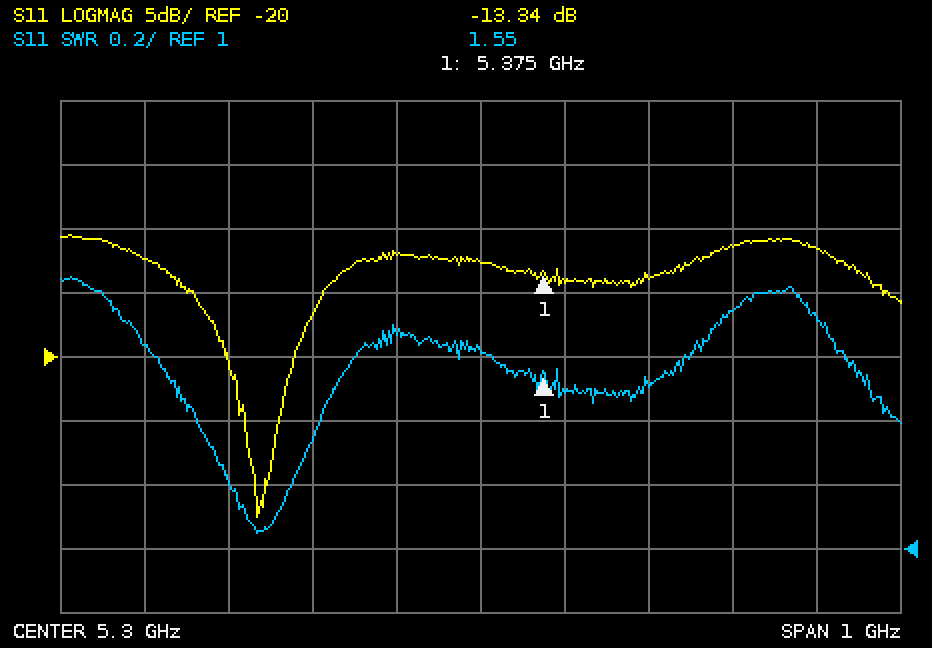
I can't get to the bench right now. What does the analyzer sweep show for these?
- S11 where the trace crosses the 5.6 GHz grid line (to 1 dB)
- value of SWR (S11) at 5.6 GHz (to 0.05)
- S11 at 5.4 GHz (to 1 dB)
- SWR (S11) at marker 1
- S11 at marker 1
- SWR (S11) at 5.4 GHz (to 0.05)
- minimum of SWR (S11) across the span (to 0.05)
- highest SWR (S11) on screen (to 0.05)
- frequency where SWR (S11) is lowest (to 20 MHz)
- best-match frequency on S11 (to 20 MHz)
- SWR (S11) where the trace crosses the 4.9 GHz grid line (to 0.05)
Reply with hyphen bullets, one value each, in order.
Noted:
- -11 dB
- 1.75
- -14 dB
- 1.55
- -13.34 dB
- 1.50
- 1.05
- 1.85
- 5.04 GHz
- 5.04 GHz
- 1.65
